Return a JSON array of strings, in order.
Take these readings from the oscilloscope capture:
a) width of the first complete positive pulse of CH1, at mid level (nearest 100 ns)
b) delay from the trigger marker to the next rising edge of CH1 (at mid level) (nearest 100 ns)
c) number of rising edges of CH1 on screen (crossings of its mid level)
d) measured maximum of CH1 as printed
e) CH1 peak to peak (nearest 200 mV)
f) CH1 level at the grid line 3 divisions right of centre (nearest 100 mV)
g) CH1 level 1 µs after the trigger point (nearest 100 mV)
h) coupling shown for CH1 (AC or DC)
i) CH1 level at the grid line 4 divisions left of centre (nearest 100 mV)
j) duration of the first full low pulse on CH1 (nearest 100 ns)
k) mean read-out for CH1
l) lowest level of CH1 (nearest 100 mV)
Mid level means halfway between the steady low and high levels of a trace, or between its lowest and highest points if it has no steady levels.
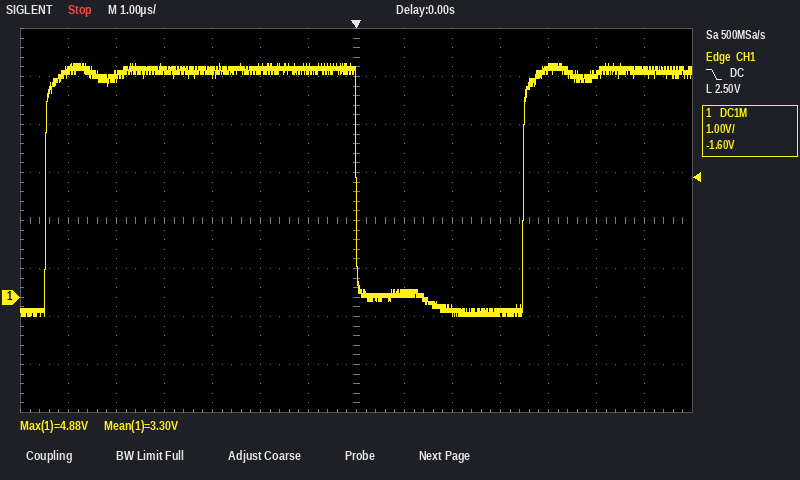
["6.5 µs", "3.5 µs", "2", "4.88 V", "5.2 V", "-300 mV", "100 mV", "DC", "4.7 V", "3.5 µs", "3.30 V", "-400 mV"]
